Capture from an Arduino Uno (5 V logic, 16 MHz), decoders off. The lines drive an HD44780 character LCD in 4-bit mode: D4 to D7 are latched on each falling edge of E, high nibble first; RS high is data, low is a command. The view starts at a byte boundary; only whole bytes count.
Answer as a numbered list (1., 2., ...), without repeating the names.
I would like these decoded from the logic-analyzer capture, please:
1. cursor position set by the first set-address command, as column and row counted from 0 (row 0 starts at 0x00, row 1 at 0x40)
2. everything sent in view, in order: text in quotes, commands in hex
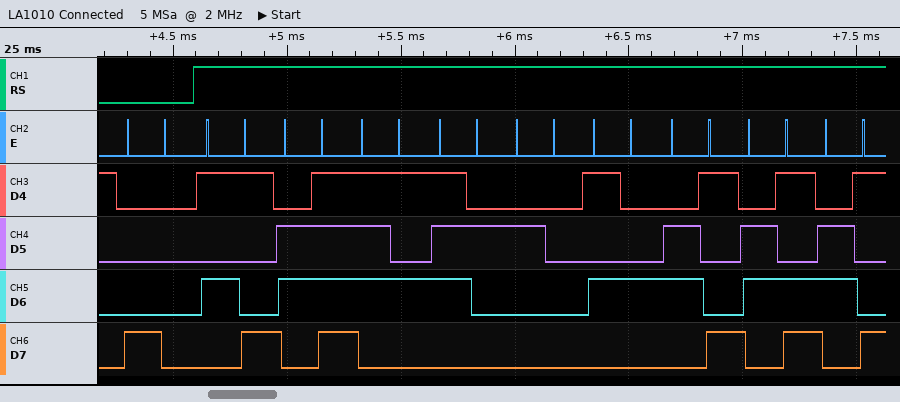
1. column 0, row 0
2. 0x80 "Your Timi"
